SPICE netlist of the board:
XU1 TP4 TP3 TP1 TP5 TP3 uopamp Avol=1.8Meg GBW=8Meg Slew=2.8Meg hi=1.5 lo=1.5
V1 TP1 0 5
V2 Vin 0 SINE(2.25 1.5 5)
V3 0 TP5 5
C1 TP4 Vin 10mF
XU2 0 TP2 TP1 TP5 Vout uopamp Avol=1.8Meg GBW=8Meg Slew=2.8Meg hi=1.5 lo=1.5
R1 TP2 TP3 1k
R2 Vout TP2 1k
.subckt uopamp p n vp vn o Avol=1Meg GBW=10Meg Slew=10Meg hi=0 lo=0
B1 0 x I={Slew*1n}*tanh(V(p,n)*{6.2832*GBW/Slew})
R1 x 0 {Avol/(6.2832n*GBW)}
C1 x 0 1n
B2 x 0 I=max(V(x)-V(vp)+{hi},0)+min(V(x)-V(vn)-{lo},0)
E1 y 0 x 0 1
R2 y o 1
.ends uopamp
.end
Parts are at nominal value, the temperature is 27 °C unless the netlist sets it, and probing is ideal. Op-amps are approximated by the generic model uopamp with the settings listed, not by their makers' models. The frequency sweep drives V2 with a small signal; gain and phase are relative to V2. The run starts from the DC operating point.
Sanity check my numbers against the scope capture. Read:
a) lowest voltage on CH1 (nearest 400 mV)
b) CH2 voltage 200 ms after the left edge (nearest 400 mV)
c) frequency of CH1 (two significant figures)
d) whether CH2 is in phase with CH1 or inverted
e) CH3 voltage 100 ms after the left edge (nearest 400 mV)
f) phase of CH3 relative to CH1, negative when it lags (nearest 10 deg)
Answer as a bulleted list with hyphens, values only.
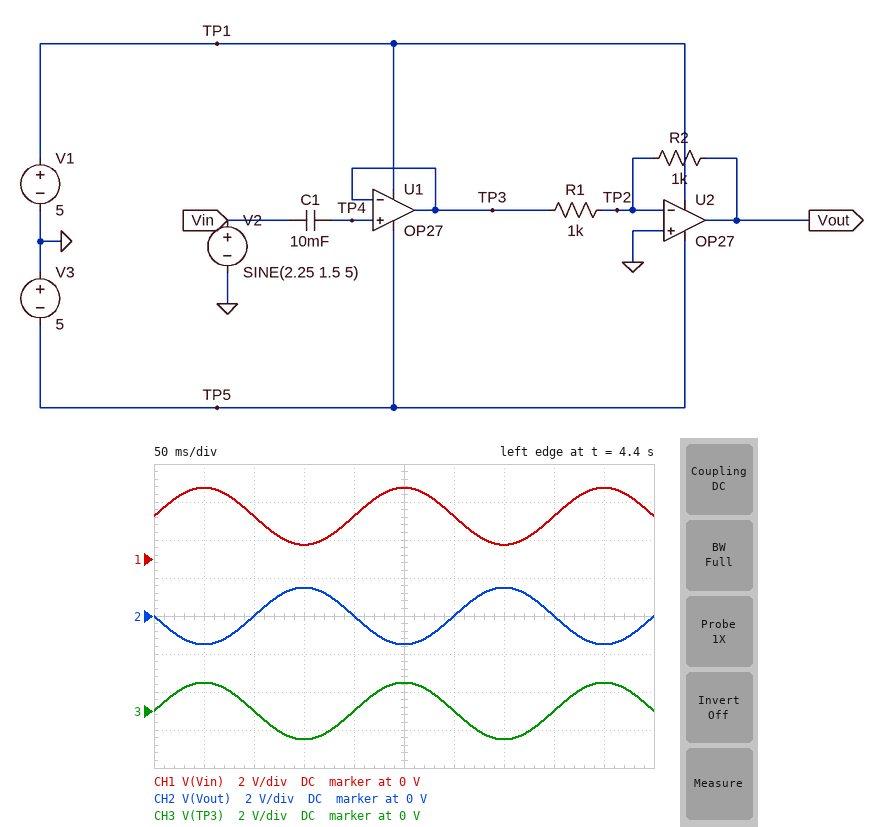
- 800 mV
- 0 V
- 5.0 Hz
- inverted
- 0 V
- 0 deg
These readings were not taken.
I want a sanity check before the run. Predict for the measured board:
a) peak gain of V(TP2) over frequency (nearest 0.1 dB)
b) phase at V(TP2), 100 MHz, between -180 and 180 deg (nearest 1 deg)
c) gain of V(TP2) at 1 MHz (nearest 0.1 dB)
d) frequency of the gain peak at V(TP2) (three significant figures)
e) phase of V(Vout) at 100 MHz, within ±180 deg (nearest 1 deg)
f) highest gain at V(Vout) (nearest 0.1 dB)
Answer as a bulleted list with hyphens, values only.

- -9.5 dB
- -83 deg
- -18.4 dB
- 5.65 MHz
- 6 deg
- 0 dB
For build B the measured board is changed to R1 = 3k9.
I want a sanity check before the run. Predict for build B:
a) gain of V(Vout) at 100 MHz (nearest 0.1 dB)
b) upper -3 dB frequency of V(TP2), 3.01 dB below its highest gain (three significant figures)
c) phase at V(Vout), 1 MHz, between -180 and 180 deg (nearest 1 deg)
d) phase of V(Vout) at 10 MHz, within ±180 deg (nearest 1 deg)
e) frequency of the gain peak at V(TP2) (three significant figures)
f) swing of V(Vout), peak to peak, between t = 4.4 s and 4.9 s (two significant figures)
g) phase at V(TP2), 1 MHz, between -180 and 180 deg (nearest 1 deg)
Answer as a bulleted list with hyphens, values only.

- -57.7 dB
- 17.3 MHz
- 164 deg
- 71 deg
- 7.14 MHz
- 770 mV
- 74 deg
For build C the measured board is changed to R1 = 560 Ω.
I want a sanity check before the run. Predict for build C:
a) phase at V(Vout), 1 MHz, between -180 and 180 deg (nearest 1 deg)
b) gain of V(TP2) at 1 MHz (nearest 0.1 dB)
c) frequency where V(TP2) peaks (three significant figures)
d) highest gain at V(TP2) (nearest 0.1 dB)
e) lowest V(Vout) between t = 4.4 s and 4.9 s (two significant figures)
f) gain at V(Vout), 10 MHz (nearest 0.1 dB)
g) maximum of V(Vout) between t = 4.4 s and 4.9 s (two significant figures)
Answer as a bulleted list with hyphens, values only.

- 154 deg
- -13.6 dB
- 4.79 MHz
- -6.5 dB
- -2.7 V
- -10.2 dB
- 2.7 V
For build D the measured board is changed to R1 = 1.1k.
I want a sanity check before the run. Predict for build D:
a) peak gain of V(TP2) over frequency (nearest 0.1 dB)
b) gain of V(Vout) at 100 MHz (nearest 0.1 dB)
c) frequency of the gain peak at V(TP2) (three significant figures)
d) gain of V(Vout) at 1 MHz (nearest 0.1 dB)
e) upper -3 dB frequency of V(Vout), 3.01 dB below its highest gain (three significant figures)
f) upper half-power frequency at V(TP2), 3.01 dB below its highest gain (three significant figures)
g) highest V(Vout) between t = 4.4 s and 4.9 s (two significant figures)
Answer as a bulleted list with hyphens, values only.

- -10.1 dB
- -50.4 dB
- 5.79 MHz
- -1.1 dB
- 3.46 MHz
- 14.5 MHz
- 1.4 V
